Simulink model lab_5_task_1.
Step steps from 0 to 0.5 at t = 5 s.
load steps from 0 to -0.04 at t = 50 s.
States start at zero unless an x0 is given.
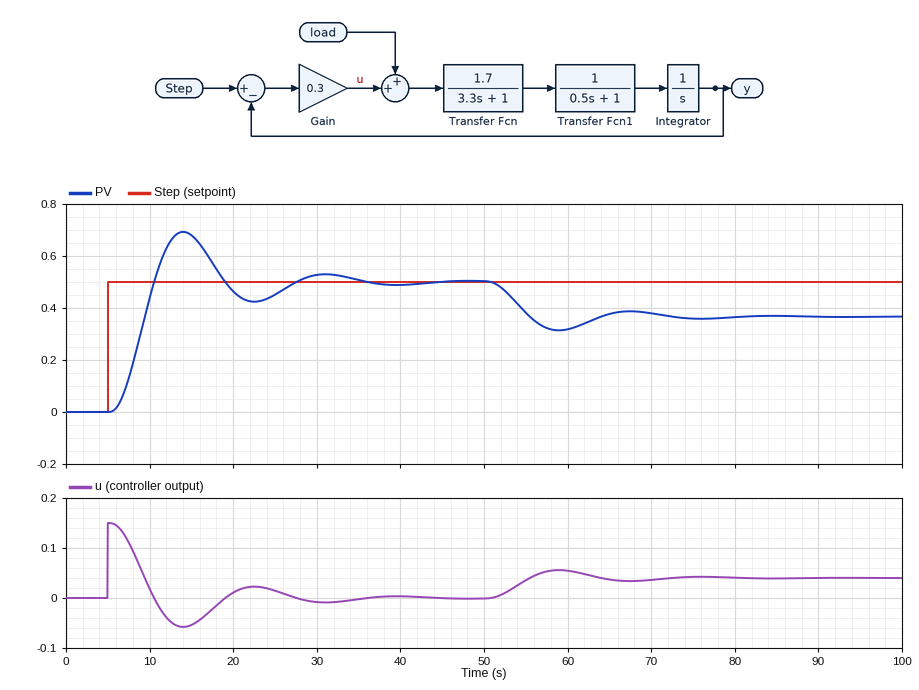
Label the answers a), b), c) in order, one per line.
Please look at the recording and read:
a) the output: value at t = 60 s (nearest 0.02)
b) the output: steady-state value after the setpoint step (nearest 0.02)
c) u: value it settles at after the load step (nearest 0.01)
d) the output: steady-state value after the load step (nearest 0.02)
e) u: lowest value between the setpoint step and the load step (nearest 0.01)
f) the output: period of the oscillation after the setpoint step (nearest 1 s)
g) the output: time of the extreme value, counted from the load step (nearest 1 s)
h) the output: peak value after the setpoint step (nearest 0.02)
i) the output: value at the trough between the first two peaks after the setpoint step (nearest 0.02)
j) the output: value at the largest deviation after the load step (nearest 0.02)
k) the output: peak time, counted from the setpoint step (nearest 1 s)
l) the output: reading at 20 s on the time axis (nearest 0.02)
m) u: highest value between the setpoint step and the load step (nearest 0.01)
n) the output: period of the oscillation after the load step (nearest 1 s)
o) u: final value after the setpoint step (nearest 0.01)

a) 0.32
b) 0.50
c) 0.04
d) 0.36
e) -0.06
f) 17 s
g) 9 s
h) 0.70
i) 0.42
j) 0.32
k) 9 s
l) 0.46
m) 0.15
n) 17 s
o) 0.00
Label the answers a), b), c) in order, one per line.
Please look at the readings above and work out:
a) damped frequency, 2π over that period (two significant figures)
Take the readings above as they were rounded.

a) 0.37 rad/s
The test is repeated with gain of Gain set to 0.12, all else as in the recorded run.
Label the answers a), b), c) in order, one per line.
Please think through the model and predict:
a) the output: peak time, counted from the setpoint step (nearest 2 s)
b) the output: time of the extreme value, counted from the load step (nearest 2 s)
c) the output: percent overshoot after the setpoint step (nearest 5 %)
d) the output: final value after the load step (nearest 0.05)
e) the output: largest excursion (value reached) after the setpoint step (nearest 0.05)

a) 16 s
b) 16 s
c) 15 %
d) 0.15
e) 0.55
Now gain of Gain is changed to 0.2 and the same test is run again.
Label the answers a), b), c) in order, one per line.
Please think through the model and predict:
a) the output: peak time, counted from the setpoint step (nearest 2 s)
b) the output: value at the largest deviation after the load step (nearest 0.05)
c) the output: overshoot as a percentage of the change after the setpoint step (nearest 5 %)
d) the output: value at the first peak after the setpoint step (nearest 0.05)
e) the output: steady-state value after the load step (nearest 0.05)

a) 12 s
b) 0.25
c) 25 %
d) 0.65
e) 0.30
